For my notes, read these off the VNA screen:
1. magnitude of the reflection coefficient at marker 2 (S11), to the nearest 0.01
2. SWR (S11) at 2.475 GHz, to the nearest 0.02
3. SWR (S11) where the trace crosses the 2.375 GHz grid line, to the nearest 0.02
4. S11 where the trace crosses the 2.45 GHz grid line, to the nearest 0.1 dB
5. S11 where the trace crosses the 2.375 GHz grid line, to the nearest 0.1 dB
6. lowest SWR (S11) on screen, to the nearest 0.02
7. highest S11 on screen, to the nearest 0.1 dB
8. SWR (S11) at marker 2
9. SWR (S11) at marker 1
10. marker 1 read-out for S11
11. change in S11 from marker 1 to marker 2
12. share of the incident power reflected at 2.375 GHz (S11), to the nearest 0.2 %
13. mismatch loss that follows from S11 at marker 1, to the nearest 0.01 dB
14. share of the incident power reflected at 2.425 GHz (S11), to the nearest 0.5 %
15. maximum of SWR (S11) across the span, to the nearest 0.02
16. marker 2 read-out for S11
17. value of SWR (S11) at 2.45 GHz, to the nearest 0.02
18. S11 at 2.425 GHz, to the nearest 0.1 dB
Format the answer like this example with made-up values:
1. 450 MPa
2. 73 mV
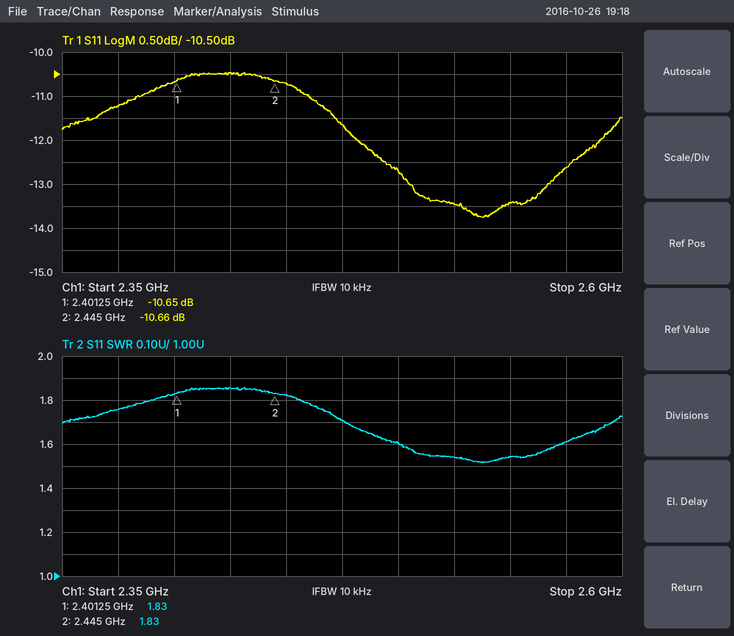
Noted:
1. 0.29
2. 1.70
3. 1.76
4. -10.7 dB
5. -11.2 dB
6. 1.52
7. -10.5 dB
8. 1.83
9. 1.83
10. -10.65 dB
11. -0.01 dB
12. 7.6 %
13. 0.39 dB
14. 9.0 %
15. 1.86
16. -10.66 dB
17. 1.82
18. -10.5 dB
